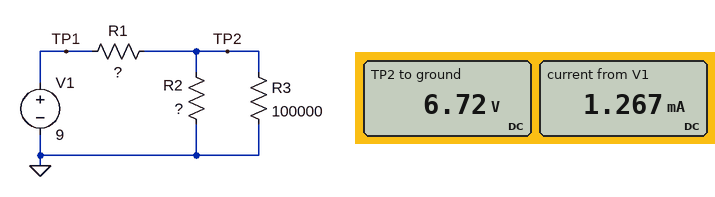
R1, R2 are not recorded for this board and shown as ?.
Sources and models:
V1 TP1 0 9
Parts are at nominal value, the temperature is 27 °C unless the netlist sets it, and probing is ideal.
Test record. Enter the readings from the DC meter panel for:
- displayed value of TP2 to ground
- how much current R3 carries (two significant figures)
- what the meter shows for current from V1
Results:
6.72 V
67 µA
1.267 mA
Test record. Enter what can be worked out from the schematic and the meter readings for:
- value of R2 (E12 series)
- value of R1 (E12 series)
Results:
5.6 kΩ
1.8 kΩ
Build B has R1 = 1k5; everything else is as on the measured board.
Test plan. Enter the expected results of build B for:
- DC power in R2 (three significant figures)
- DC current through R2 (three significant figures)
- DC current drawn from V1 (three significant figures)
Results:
8.79 mW
1.25 mA
1.32 mA
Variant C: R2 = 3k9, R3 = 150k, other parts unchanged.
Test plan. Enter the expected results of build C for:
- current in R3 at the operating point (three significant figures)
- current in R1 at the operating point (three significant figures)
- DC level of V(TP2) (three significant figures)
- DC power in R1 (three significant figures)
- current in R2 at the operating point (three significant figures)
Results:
40.7 µA
1.61 mA
6.11 V
4.65 mW
1.57 mA
